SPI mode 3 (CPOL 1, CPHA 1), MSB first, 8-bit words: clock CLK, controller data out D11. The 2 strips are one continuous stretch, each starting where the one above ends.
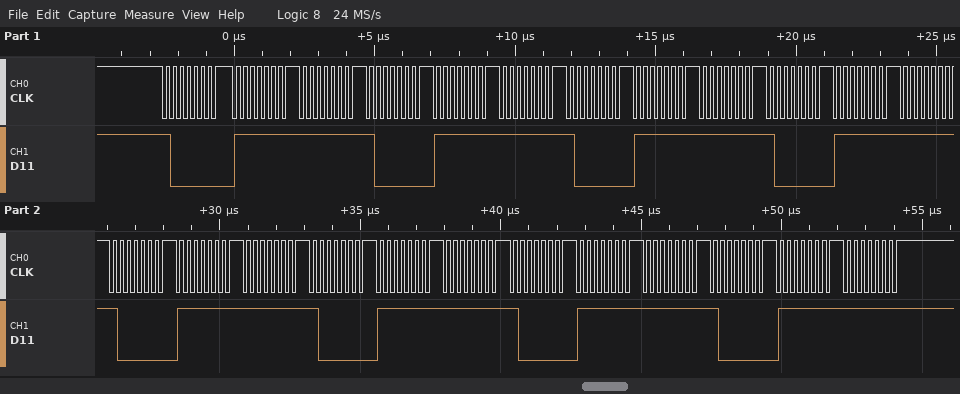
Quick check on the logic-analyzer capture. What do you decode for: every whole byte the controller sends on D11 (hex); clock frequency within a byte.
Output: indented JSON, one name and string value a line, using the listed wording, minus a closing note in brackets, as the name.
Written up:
{
  "every whole byte the controller sends on D11": "80 FF FF 80 FF FF 80 FF FF 80 FF FF 80 FF FF 80 FF FF 80 FF FF 80 FF FF",
  "clock frequency within a byte": "4 MHz"
}
